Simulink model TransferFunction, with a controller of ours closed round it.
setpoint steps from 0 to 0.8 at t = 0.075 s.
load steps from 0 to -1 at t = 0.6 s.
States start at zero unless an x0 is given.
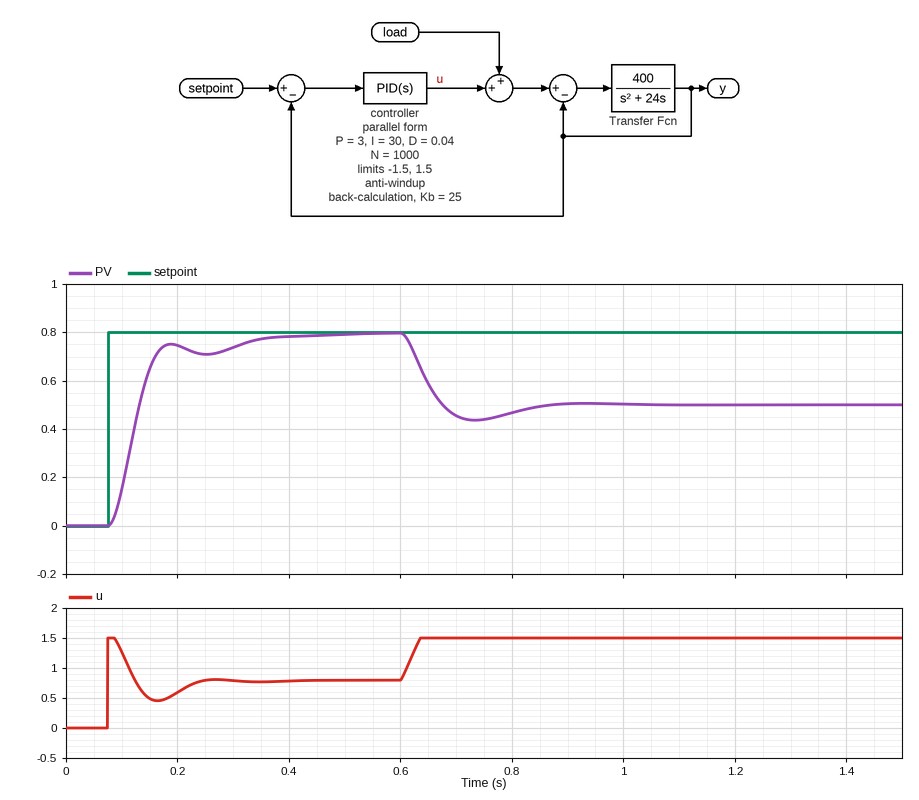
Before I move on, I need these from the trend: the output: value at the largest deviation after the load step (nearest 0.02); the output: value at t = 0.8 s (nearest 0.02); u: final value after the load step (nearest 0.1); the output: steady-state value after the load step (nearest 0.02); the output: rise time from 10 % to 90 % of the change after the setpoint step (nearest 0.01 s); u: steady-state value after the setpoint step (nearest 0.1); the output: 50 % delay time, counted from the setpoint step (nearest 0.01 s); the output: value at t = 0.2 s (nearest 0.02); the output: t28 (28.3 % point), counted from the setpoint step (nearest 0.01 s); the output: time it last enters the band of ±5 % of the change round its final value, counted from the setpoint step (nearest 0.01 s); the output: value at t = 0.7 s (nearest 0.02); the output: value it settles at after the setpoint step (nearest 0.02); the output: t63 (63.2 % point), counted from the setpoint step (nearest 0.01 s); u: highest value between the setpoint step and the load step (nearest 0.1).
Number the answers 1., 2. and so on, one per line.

1. 0.44
2. 0.46
3. 1.5
4. 0.50
5. 0.07 s
6. 0.8
7. 0.05 s
8. 0.74
9. 0.03 s
10. 0.25 s
11. 0.46
12. 0.80
13. 0.06 s
14. 1.5
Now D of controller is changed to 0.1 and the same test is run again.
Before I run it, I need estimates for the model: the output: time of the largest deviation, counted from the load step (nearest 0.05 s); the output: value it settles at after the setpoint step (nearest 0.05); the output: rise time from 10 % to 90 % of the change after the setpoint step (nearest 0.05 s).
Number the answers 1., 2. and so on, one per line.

1. 0.15 s
2. 0.80
3. 0.20 s
